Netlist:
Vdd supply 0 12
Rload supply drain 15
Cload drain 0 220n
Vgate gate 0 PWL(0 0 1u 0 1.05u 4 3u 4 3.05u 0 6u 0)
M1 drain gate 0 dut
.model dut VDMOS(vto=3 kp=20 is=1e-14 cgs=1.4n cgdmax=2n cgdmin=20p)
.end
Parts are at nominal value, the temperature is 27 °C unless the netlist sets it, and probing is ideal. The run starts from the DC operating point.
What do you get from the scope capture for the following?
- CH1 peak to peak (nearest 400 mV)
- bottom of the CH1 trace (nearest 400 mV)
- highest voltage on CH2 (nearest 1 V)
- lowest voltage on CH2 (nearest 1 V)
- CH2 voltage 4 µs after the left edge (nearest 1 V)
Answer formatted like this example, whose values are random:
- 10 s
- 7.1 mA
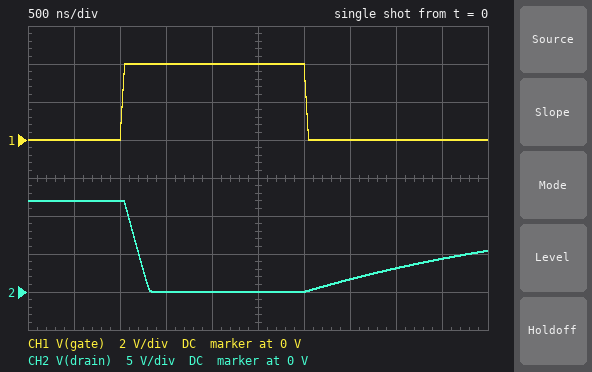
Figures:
- 4.0 V
- 0 V
- 12 V
- 0 V
- 3 V
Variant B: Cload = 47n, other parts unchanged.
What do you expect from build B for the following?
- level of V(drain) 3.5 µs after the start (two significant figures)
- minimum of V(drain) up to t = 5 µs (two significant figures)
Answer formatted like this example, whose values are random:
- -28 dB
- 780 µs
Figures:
- 5.9 V
- 38 mV
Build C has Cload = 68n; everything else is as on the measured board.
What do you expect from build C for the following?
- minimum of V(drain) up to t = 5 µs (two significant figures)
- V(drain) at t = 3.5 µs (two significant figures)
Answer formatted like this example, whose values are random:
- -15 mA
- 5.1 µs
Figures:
- 39 mV
- 4.5 V
